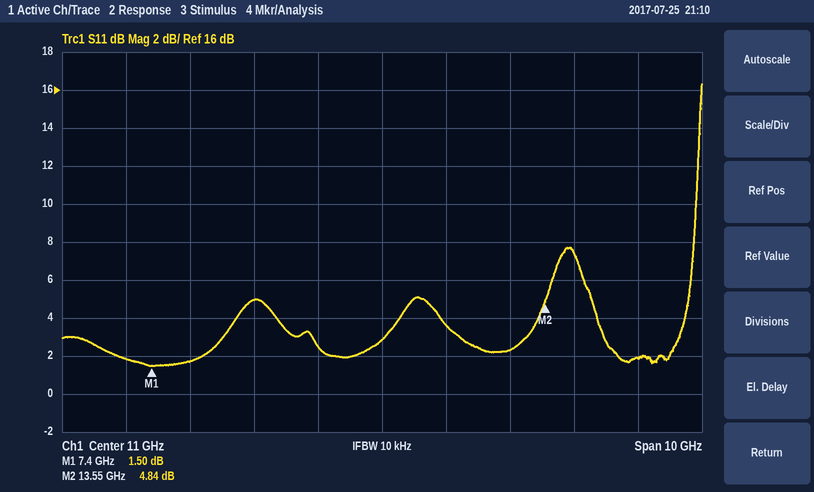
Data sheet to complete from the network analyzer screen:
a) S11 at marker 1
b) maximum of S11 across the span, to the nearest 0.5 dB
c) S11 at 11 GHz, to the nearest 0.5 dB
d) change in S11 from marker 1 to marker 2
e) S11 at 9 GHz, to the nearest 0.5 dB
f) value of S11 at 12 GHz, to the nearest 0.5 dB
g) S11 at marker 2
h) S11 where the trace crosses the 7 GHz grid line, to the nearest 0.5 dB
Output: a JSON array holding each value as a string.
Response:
["1.50 dB", "16.5 dB", "3.0 dB", "3.34 dB", "5.0 dB", "3.5 dB", "4.84 dB", "2.0 dB"]
